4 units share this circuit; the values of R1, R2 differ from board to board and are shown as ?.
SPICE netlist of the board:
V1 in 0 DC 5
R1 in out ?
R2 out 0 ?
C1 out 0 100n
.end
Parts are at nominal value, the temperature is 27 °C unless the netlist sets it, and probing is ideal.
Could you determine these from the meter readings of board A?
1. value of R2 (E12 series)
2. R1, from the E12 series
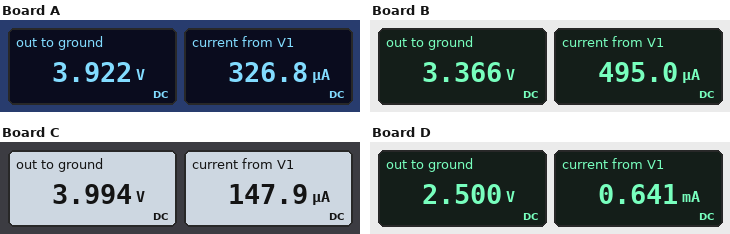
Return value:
12 kΩ
3.3 kΩ
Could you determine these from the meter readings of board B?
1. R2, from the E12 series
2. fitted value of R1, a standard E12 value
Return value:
6.8 kΩ
3.3 kΩ
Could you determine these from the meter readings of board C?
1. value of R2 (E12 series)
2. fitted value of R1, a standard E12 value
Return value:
27 kΩ
6.8 kΩ
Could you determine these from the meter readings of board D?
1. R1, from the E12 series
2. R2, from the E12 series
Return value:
3.9 kΩ
3.9 kΩ
